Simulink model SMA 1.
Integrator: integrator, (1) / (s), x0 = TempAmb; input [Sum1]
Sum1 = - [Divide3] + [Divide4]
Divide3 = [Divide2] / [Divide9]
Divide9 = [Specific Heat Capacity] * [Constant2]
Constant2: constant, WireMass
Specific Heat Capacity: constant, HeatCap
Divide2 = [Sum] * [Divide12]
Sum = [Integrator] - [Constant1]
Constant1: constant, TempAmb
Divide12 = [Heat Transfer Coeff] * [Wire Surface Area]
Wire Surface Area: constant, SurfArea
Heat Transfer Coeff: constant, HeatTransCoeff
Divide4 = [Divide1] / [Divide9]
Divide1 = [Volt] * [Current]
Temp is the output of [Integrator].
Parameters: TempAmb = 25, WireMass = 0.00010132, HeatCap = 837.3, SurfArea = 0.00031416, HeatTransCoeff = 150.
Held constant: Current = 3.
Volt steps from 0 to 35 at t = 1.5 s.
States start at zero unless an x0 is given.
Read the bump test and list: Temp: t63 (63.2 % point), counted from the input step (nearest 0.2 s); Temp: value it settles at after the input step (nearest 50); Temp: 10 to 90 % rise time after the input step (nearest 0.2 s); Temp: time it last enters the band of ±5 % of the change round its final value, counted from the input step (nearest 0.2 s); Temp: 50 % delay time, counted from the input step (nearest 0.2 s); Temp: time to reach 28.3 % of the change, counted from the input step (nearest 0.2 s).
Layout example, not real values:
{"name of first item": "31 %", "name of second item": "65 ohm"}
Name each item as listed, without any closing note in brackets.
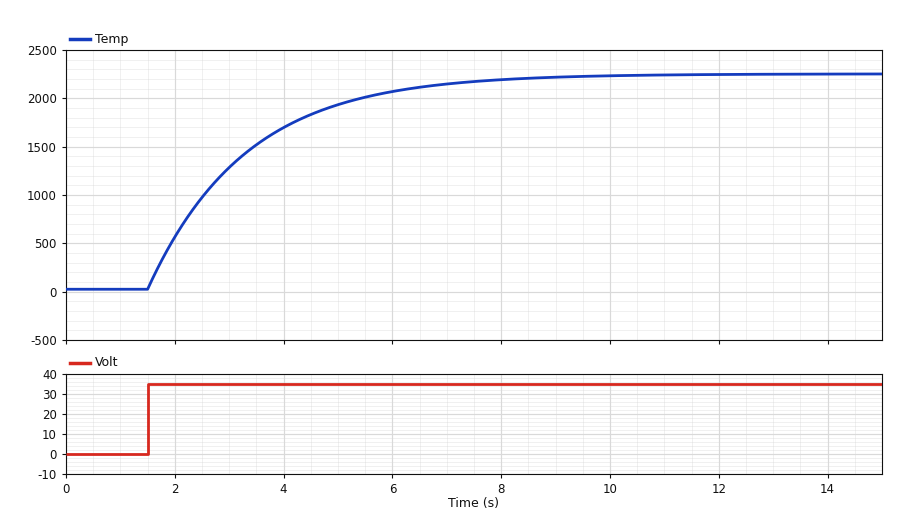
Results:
{"Temp: t63 (63.2 % point), counted from the input step": "1.8 s", "Temp: value it settles at after the input step": "2250", "Temp: 10 to 90 % rise time after the input step": "4.0 s", "Temp: time it last enters the band of ±5 % of the change round its final value, counted from the input step": "5.4 s", "Temp: 50 % delay time, counted from the input step": "1.2 s", "Temp: time to reach 28.3 % of the change, counted from the input step": "0.6 s"}
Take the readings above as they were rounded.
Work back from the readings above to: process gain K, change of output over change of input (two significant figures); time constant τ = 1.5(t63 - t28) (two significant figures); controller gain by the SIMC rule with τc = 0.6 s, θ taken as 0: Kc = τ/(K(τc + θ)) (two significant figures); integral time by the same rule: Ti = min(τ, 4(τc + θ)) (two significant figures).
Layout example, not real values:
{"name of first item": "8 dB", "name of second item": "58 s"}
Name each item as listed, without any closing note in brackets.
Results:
{"process gain K, change of output over change of input": "64", "time constant τ = 1.5(t63 - t28)": "1.8 s", "controller gain by the SIMC rule with τc = 0.6 s, θ taken as 0: Kc = τ/(K(τc + θ))": "0.047", "integral time by the same rule: Ti = min(τ, 4(τc + θ))": "1.8 s"}
